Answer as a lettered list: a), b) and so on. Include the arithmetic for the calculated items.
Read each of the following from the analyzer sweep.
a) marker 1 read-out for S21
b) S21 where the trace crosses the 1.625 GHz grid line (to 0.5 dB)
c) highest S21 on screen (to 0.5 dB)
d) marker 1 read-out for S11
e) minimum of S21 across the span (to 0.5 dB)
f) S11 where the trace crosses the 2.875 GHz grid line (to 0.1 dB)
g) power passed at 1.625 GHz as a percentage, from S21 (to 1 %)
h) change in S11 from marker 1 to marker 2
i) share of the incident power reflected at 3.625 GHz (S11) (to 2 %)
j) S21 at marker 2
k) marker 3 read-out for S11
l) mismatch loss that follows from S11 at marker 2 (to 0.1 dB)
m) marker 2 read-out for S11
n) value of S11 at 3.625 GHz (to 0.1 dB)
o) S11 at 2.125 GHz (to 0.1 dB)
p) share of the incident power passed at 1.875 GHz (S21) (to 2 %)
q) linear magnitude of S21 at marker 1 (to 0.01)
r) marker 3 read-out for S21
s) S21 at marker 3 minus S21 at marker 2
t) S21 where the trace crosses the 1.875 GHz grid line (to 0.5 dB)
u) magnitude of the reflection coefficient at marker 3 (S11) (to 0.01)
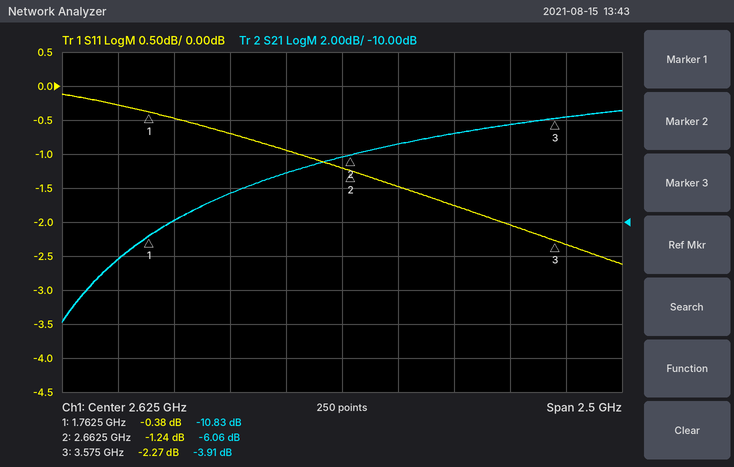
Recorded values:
a) -10.83 dB
b) -12.0 dB
c) -3.5 dB
d) -0.38 dB
e) -16.0 dB
f) -1.5 dB
g) 10^(-12/10) ≈ 6 %
h) -1.24 − (-0.38) = -0.86 dB
i) 10^(-2.3/10) ≈ 58.9 %, so 58 % to the nearest 2 %
j) -6.06 dB
k) -2.27 dB
l) −10 log10(1 − 10^(-1.24/10)) ≈ 6.0 dB
m) -1.24 dB
n) -2.3 dB
o) -0.7 dB
p) 10^(-10/10) ≈ 10 %
q) 10^(-10.83/20) ≈ 0.29
r) -3.91 dB
s) -3.91 − (-6.06) = 2.15 dB
t) -10.0 dB
u) 10^(-2.27/20) ≈ 0.77
